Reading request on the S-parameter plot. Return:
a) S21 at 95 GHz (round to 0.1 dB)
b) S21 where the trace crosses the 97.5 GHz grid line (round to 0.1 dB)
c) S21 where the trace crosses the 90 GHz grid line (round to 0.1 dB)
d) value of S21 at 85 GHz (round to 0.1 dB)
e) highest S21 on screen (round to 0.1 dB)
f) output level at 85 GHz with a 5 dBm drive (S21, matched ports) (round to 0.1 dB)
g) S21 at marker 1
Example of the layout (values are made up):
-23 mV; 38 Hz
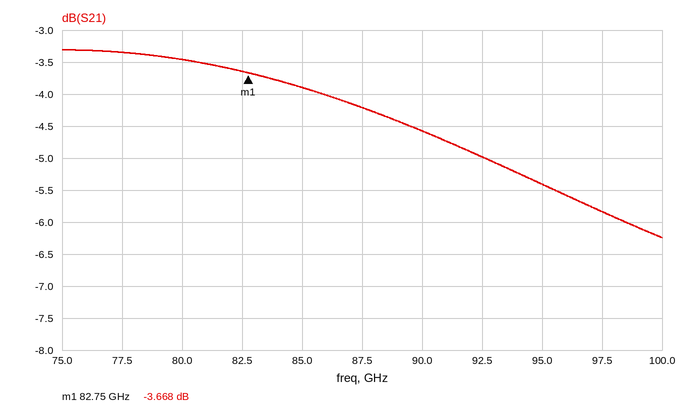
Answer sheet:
-5.4 dB; -5.8 dB; -4.6 dB; -3.9 dB; -3.3 dB; 1.1 dBm; -3.668 dB
